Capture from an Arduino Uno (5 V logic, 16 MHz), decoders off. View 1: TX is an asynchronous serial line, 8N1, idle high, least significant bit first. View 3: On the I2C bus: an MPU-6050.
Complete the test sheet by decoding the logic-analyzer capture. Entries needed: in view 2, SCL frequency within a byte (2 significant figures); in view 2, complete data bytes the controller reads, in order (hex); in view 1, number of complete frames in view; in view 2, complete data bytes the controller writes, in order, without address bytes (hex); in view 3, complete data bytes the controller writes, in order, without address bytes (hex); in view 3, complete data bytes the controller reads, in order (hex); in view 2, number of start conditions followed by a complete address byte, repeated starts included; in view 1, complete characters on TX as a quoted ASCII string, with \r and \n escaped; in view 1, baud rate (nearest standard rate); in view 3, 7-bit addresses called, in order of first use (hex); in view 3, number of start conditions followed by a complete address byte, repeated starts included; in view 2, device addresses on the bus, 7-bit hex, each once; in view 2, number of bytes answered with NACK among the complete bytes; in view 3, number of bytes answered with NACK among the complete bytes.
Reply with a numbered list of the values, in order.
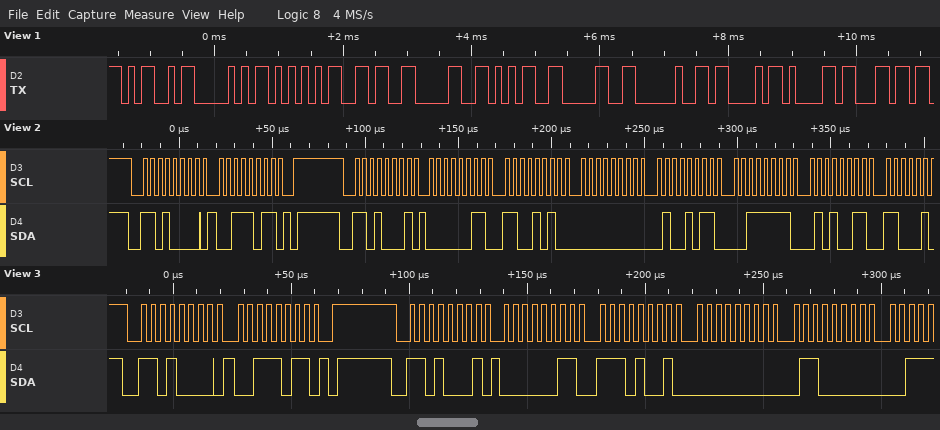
1. 250 kHz
2. 03 CA 00 4B 3F 53
3. 11
4. 3B
5. 3B
6. 03 E9 00 60
7. 2
8. "MPU6050 Cal"
9. 9600 baud
10. 0x68
11. 2
12. 0x68
13. 0
14. 0
